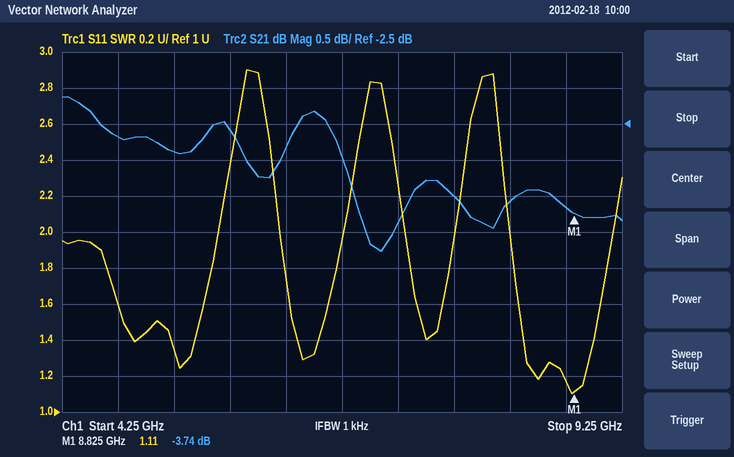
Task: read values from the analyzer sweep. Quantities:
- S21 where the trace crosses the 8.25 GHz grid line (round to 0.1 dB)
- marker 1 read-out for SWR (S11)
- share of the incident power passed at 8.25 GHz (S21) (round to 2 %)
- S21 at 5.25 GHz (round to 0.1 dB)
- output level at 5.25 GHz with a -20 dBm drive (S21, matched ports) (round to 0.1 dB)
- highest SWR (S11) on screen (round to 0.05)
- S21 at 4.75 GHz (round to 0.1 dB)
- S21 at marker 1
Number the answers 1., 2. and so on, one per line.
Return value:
1. -3.6 dB
2. 1.11
3. 44 %
4. -2.9 dB
5. -22.9 dBm
6. 2.90
7. -2.7 dB
8. -3.74 dB
